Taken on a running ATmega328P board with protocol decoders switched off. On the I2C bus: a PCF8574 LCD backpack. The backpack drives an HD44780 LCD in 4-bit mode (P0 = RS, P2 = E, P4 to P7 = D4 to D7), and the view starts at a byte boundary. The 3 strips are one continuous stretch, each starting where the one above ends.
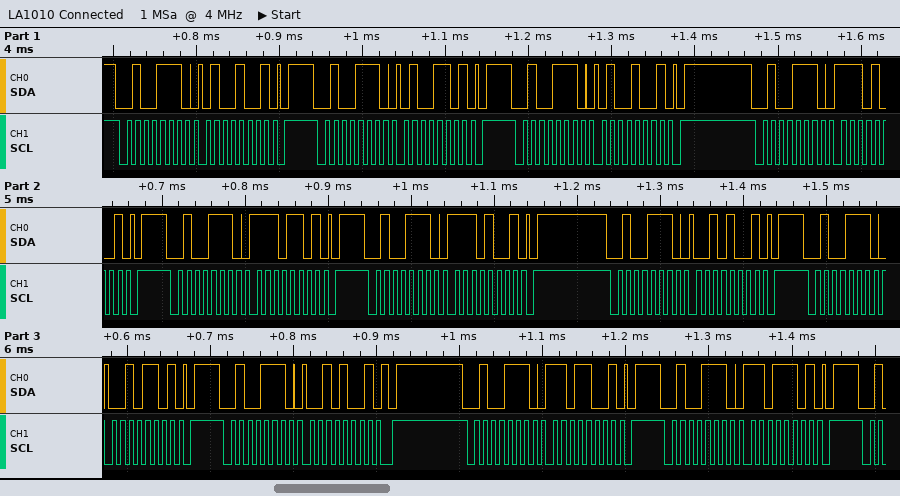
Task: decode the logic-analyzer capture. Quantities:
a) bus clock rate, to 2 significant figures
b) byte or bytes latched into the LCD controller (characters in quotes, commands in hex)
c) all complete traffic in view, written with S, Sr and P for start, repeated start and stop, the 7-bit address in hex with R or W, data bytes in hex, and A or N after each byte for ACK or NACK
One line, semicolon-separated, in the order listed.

100 kHz; 'N'; S 27W A 49 A P S 27W A 4D A P S 27W A 49 A P S 27W A E9 A P S 27W A ED A P S 27W A E9 A P S 27W A 29 A P S 27W A 2D A P S 27W A 29 A P S 27W A D9 A P S 27W A DD A P
